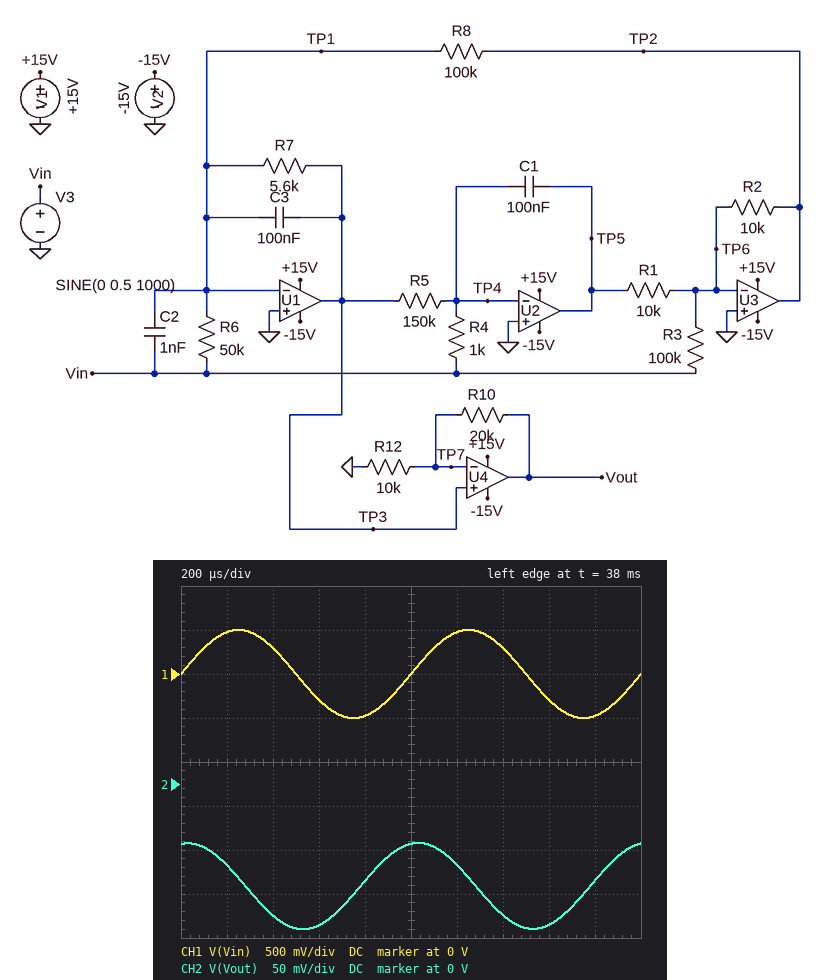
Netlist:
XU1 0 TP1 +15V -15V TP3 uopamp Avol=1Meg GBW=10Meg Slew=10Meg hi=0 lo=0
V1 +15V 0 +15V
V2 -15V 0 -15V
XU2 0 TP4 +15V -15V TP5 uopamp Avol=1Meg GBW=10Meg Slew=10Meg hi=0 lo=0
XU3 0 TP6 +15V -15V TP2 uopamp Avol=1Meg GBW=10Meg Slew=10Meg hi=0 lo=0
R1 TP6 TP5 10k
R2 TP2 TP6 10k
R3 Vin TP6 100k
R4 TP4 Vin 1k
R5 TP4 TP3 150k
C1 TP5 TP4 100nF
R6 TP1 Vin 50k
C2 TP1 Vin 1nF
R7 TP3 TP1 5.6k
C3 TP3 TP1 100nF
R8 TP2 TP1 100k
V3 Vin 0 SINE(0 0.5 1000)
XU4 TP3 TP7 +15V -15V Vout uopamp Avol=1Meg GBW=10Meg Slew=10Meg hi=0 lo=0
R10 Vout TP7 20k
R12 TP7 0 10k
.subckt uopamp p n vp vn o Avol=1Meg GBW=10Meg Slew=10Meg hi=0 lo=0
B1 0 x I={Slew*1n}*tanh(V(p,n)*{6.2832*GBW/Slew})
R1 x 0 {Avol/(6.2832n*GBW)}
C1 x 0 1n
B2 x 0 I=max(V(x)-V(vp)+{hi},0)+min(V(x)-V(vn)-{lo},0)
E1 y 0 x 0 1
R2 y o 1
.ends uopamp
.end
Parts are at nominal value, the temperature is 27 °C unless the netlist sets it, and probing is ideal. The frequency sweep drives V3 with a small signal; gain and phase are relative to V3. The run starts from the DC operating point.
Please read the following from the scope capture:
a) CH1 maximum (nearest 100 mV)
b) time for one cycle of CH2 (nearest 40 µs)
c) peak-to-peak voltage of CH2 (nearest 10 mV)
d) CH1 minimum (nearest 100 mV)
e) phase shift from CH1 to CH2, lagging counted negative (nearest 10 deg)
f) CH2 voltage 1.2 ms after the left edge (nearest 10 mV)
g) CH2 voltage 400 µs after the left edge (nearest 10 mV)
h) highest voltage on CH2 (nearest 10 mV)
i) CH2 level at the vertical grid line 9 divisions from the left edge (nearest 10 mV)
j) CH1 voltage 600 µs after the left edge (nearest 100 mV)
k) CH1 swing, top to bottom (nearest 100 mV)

500 mV
1.00 ms
100 mV
-500 mV
80 deg
-90 mV
-150 mV
-70 mV
-110 mV
-300 mV
1.0 V
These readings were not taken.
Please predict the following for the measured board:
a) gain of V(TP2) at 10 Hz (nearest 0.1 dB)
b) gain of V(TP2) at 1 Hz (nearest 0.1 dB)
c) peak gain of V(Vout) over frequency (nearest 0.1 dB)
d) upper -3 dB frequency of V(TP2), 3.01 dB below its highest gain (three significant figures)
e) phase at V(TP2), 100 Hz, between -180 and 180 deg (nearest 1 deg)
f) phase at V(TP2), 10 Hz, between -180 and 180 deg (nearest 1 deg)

44.0 dB
62.7 dB
53.0 dB
597 mHz
-90 deg
-87 deg
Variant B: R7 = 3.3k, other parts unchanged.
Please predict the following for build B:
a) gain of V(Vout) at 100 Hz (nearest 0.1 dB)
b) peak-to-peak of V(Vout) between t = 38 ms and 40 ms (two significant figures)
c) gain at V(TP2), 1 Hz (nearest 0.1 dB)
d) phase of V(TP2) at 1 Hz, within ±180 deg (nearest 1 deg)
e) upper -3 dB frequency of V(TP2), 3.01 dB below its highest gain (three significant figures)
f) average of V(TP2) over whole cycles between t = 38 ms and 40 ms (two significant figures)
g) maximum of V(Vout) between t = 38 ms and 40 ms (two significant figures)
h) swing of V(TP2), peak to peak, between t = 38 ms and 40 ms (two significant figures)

3.8 dB
92 mV
63.5 dB
-71 deg
352 mHz
730 mV
-26 mV
1.6 V
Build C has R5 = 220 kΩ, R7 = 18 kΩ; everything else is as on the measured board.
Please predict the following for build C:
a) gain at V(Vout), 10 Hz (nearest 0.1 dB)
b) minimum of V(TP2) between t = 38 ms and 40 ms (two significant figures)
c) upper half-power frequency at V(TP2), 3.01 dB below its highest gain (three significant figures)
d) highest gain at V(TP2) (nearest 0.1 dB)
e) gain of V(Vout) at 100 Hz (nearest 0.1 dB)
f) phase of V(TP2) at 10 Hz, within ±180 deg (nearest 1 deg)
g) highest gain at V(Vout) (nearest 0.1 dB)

38.7 dB
-220 mV
1.32 Hz
61.7 dB
15.2 dB
-83 deg
56.4 dB
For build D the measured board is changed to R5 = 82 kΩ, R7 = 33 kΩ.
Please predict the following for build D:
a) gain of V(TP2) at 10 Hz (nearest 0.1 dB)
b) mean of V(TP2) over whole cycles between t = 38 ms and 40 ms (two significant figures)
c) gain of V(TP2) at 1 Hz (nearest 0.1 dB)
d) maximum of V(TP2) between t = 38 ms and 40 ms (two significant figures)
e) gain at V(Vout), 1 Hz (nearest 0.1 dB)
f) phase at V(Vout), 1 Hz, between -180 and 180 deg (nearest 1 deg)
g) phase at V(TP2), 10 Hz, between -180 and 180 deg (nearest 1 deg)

43.4 dB
150 mV
47.8 dB
950 mV
47.7 dB
171 deg
-55 deg
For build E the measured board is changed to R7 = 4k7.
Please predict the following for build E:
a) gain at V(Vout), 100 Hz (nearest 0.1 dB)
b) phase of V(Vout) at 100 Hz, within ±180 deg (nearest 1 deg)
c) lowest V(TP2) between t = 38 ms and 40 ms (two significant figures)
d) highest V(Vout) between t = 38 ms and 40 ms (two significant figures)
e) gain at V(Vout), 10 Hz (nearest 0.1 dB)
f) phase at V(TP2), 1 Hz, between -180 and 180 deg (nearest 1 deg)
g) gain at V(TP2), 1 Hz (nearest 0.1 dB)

6.7 dB
81 deg
-94 mV
-51 mV
27.0 dB
-63 deg
63.1 dB
